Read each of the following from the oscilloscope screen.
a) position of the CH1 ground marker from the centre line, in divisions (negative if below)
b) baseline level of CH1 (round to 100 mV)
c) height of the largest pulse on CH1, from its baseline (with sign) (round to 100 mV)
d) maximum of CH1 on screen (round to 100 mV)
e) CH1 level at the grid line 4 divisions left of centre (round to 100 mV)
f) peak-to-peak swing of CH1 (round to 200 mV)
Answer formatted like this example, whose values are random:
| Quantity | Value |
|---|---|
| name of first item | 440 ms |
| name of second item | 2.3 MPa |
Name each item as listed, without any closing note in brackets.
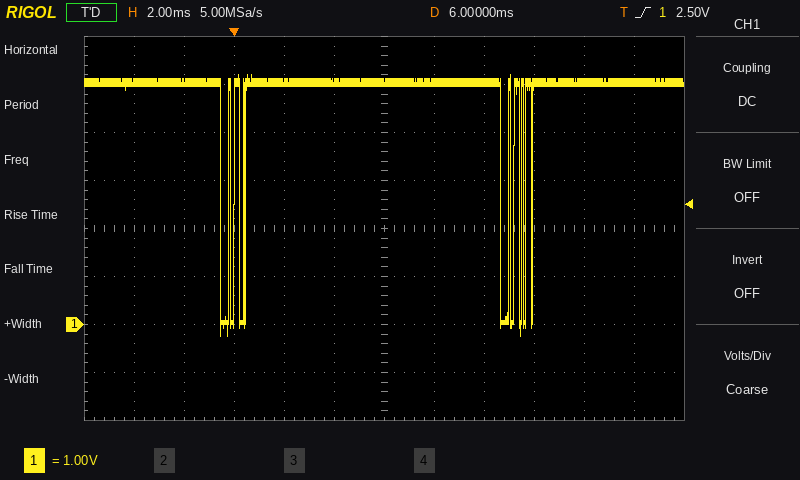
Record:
| Quantity | Value |
|---|---|
| position of the CH1 ground marker from the centre line, in divisions | -2.0 div |
| baseline level of CH1 | 5.0 V |
| height of the largest pulse on CH1, from its baseline (with sign) | -5.3 V |
| maximum of CH1 on screen | 5.2 V |
| CH1 level at the grid line 4 divisions left of centre | 5.0 V |
| peak-to-peak swing of CH1 | 5.4 V |
